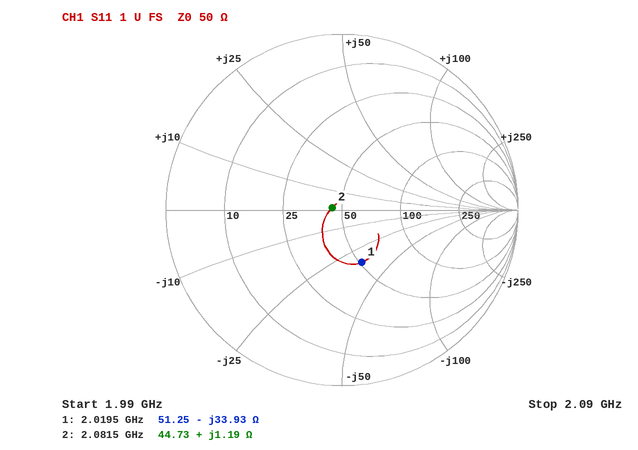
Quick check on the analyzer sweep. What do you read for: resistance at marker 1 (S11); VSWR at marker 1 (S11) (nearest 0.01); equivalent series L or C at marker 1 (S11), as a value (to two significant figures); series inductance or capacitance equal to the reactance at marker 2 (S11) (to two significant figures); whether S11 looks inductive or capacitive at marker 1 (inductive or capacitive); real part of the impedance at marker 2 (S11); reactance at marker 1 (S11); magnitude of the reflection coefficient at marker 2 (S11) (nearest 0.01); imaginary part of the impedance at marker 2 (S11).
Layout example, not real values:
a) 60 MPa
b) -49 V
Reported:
a) 51.25 Ω
b) 1.93
c) 2.3 pF
d) 91 pH
e) capacitive
f) 44.73 Ω
g) -33.93 Ω
h) 0.06
i) +1.19 Ω
